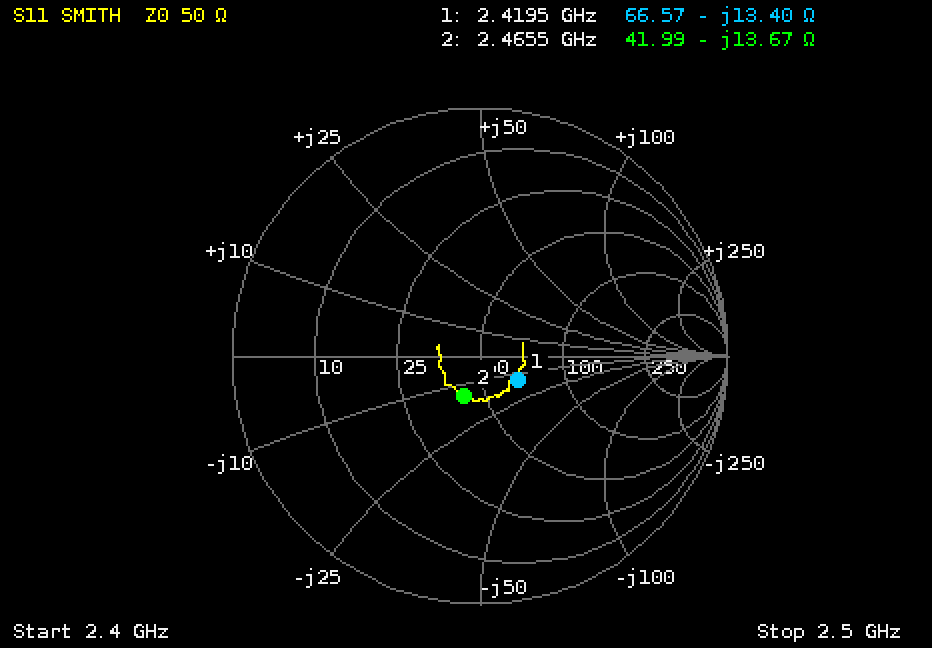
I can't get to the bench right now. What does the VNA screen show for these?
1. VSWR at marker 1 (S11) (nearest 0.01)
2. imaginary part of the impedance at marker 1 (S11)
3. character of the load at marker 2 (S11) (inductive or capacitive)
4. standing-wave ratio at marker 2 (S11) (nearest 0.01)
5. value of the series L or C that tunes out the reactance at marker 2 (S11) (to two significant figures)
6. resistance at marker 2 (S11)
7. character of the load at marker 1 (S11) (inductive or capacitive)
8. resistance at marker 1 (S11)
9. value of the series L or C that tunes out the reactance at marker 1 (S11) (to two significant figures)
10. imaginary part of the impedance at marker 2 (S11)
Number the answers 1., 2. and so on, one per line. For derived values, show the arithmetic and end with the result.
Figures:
1. 1.44
2. -13.40 Ω
3. capacitive
4. 1.41
5. L = 13.67 Ω/(2π × 2.4655 GHz) ≈ 882 pH, so 880 pH to two significant figures
6. 41.99 Ω
7. capacitive
8. 66.57 Ω
9. L = 13.4 Ω/(2π × 2.4195 GHz) ≈ 881 pH, so 880 pH to two significant figures
10. -13.67 Ω
